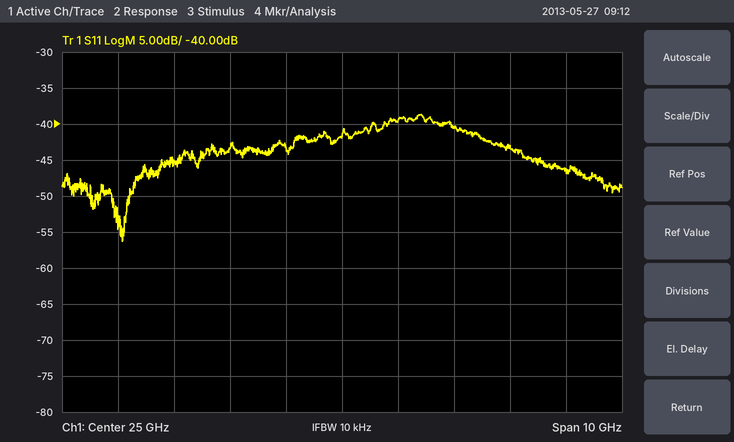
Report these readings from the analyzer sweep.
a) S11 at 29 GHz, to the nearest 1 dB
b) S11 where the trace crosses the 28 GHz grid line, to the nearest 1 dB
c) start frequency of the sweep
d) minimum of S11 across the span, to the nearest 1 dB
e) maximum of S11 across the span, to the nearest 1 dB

-46 dB
-43 dB
20 GHz
-56 dB
-39 dB
